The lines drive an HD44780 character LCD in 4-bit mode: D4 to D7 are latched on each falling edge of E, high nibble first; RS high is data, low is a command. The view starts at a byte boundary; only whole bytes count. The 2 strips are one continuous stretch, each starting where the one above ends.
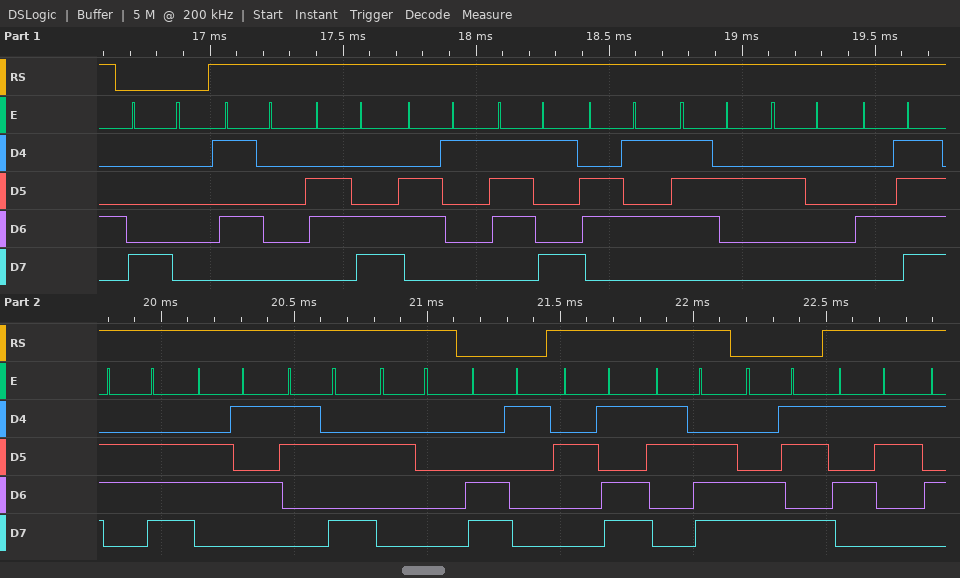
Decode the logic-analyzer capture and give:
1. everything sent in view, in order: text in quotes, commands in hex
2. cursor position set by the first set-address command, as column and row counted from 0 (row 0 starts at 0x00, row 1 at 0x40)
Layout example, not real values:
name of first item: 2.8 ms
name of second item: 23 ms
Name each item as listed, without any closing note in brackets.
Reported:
everything sent in view, in order: text in quotes, commands in hex: 0x80 "Player One: " 0xC1 "->" 0xCB "S"
cursor position set by the first set-address command, as column and row counted from 0: column 0, row 0
